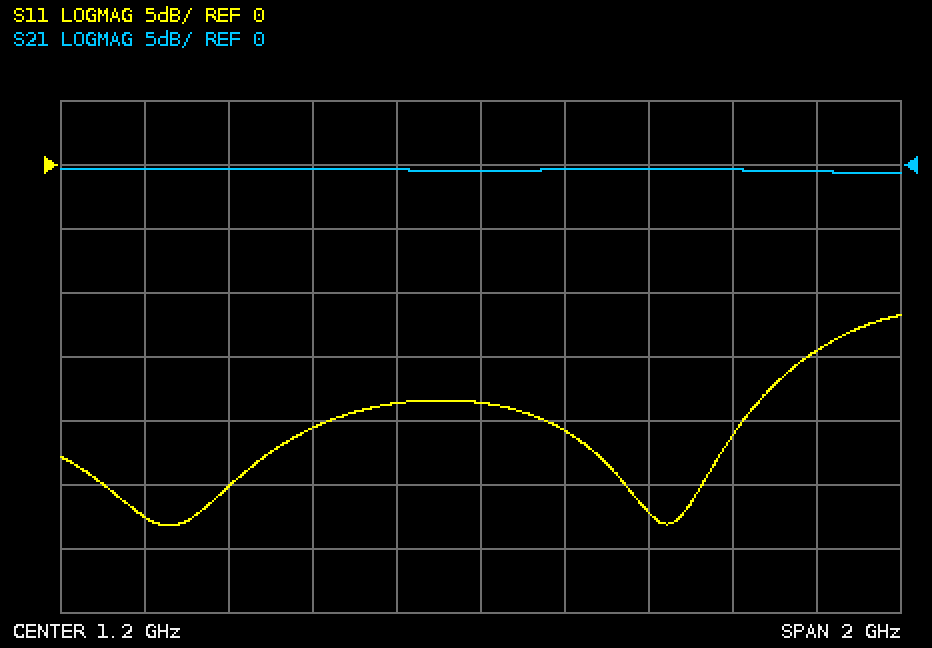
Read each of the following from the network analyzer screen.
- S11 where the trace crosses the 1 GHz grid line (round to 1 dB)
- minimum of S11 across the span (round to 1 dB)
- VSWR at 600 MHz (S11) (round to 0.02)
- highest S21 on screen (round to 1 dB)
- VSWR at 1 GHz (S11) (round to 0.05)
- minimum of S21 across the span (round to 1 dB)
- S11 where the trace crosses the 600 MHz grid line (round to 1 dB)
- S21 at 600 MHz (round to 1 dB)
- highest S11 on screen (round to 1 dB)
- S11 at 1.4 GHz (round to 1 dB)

-19 dB
-28 dB
1.12
0 dB
1.25
-1 dB
-25 dB
0 dB
-12 dB
-21 dB
